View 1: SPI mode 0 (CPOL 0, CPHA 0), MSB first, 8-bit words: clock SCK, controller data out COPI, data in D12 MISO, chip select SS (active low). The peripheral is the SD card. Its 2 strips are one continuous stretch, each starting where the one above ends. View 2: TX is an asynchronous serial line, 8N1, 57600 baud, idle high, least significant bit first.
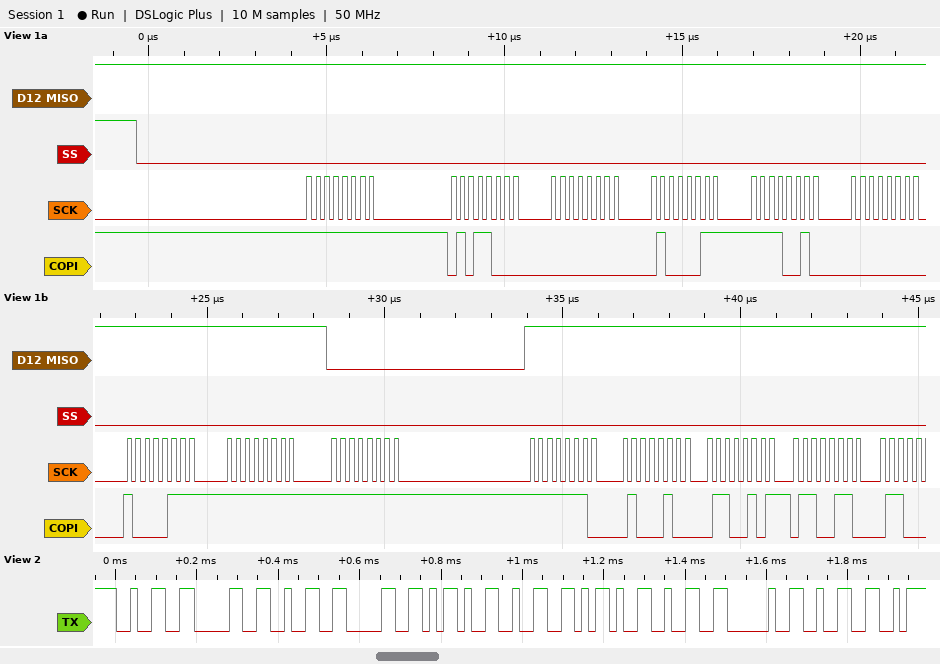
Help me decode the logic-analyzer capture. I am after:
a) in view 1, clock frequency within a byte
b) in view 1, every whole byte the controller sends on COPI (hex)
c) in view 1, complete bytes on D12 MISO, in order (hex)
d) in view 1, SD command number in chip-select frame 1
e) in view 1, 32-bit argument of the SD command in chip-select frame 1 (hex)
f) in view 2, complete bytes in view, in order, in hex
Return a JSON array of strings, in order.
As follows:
["4 MHz", "FF 58 00 43 F2 00 87 FF FF FE 44 65 66", "FF FF FF FF FF FF FF FF 00 FF FF FF FF", "CMD24", "0x0043F200", "0x32 0x30 0x32 0x30 0x2D 0x32 0x2D 0x32 0x20 0x32"]
